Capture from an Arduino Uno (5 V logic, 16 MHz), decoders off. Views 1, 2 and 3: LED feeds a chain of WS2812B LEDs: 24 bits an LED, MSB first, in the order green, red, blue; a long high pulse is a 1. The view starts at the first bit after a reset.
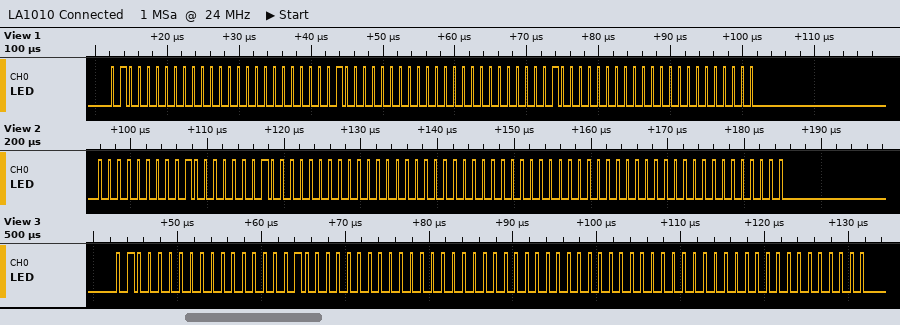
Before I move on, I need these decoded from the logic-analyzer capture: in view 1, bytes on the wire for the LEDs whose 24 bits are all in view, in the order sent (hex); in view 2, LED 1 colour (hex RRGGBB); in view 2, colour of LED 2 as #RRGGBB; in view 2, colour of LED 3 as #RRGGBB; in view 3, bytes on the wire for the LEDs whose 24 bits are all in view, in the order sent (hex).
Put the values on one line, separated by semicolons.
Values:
40 00 00 40 00 00 40 00 00; #400040; #000000; #000000; 40 00 40 00 00 00 00 00 00
